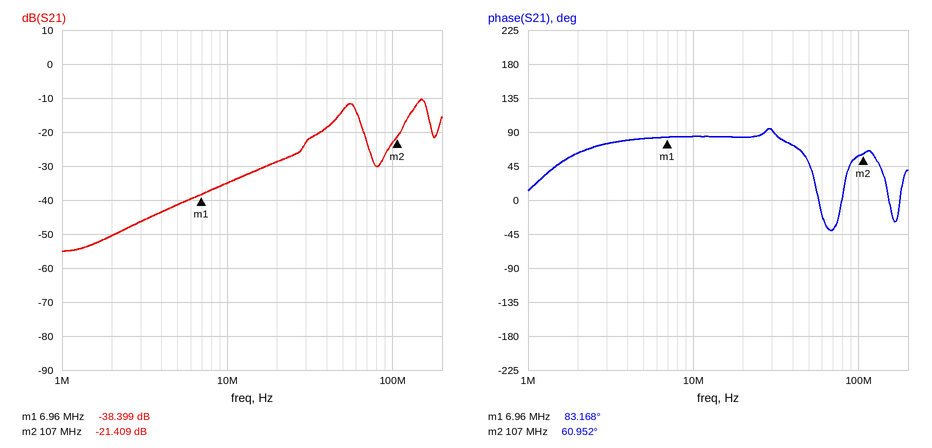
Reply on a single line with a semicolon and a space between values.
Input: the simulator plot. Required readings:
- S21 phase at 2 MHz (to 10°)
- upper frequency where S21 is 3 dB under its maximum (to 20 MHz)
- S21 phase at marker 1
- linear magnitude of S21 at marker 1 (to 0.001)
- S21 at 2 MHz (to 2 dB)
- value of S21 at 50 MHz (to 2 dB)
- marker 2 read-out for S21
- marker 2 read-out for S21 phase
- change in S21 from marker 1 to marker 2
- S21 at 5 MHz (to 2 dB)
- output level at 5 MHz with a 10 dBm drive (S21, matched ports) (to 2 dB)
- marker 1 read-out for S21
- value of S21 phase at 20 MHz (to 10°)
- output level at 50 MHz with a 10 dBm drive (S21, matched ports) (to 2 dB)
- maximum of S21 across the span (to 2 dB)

60°; 160 MHz; 83.168°; 0.012; -50 dB; -14 dB; -21.409 dB; 60.952°; 16.990 dB; -42 dB; -32 dBm; -38.399 dB; 80°; -4 dBm; -10 dB
